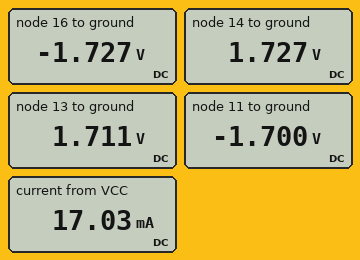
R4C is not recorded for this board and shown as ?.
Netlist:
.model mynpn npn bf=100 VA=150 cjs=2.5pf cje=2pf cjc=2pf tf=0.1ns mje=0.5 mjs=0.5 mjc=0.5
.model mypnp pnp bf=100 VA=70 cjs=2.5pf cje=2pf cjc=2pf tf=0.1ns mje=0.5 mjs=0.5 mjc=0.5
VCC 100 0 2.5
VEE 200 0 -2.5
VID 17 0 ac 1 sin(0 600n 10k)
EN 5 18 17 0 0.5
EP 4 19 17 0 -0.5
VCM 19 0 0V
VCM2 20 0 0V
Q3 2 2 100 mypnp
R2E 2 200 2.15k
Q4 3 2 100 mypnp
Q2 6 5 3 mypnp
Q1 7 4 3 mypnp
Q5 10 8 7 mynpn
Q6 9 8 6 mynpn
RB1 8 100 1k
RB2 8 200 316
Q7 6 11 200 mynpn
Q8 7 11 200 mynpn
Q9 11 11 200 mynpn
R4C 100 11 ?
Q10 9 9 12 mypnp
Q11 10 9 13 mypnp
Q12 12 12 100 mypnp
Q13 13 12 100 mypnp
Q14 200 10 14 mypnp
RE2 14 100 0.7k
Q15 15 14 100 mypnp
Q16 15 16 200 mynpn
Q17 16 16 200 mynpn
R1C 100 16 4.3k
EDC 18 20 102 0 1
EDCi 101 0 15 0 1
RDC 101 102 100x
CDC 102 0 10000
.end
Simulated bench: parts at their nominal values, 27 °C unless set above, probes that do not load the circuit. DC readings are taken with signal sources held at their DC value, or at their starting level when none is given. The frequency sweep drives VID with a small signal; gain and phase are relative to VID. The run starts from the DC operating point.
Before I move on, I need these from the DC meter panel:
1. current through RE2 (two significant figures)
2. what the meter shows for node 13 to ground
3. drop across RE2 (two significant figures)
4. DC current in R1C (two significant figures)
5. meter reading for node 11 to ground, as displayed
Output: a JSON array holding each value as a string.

["1.1 mA", "1.711 V", "770 mV", "980 µA", "-1.700 V"]
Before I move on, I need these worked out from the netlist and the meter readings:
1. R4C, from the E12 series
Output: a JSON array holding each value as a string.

["1.5 kΩ"]
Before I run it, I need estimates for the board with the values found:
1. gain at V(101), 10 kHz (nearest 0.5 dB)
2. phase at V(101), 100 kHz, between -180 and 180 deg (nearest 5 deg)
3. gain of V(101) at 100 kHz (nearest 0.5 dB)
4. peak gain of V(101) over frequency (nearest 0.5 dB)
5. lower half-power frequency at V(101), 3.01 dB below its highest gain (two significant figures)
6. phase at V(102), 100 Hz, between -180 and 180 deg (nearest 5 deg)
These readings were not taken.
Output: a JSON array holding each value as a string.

["131.5 dB", "125 deg", "128.0 dB", "131.5 dB", "610 mHz", "90 deg"]
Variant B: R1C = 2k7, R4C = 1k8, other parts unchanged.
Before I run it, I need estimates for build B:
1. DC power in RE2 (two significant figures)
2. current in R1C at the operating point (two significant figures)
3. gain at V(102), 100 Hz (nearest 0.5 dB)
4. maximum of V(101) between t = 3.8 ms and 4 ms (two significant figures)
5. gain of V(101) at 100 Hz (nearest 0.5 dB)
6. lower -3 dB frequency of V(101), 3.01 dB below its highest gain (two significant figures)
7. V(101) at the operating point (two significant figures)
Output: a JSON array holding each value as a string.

["880 µW", "1.6 mA", "-45.0 dB", "2.0 V", "131.0 dB", "550 mHz", "1.1 mV"]
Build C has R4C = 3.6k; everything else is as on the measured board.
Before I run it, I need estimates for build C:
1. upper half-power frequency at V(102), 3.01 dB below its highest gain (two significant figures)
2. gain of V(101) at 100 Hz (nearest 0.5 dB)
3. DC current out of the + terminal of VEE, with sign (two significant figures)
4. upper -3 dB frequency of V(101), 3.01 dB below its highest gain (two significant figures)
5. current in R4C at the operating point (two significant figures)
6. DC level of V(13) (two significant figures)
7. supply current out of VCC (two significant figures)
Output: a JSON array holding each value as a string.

["630 mHz", "132.0 dB", "-12 mA", "84 kHz", "1.2 mA", "1.8 V", "12 mA"]
